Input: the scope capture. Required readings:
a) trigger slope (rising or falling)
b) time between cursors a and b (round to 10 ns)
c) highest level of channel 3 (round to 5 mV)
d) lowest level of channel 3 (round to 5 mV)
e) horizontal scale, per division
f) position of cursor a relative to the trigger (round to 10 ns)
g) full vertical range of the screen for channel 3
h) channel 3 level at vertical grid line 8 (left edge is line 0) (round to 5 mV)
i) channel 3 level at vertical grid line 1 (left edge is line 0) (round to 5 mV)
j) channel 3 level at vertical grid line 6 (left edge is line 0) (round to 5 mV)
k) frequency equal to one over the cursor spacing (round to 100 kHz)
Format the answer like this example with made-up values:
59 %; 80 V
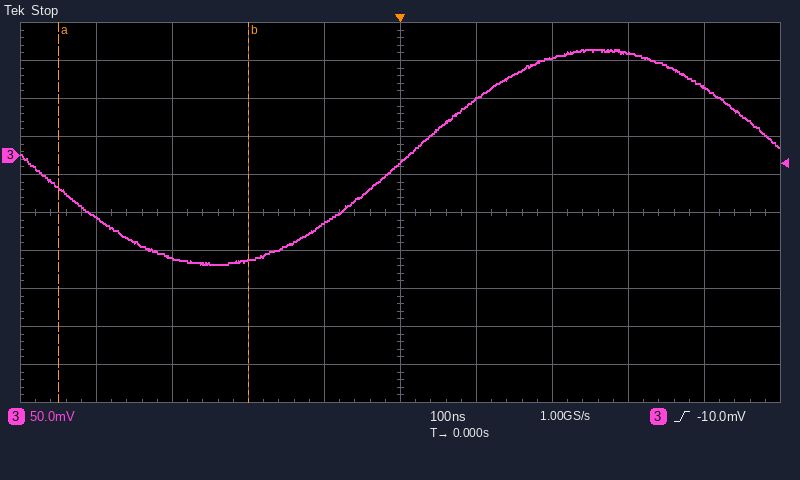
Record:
rising; 250 ns; 140 mV; -145 mV; 100 ns; -450 ns; 500 mV; 135 mV; -80 mV; 75 mV; 4.0 MHz
